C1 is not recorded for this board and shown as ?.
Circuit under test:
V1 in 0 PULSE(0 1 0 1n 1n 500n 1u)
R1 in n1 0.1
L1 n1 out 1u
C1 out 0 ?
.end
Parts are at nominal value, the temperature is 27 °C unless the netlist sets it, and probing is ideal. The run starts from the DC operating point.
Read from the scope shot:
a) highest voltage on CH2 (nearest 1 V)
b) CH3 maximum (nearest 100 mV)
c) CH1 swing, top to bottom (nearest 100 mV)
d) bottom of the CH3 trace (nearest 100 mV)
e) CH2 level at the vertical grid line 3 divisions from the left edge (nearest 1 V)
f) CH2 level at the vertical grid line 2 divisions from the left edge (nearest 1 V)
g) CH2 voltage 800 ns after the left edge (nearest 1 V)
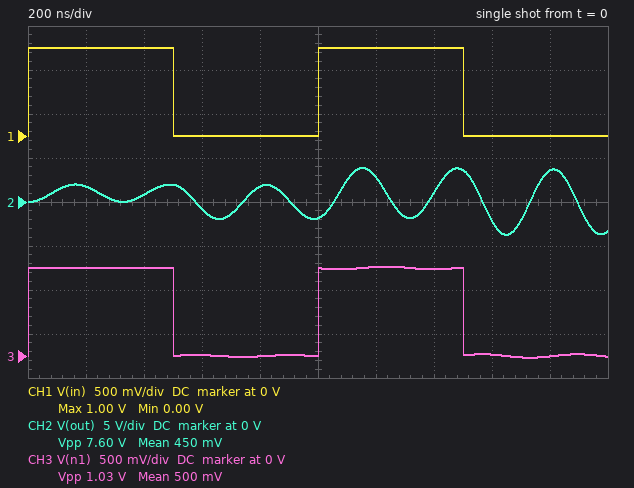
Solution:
4 V
1.0 V
1.0 V
0 V
-1 V
1 V
2 V
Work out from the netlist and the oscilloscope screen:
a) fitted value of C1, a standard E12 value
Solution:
2.7 nF
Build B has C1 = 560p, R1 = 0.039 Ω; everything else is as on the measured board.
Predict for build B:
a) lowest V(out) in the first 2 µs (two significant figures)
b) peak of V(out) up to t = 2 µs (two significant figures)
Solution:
-2.3 V
3.3 V
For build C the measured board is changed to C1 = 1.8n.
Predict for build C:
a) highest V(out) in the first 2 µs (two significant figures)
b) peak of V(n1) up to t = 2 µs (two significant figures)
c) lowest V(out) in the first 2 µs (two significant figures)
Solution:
2.0 V
1.0 V
-1.0 V
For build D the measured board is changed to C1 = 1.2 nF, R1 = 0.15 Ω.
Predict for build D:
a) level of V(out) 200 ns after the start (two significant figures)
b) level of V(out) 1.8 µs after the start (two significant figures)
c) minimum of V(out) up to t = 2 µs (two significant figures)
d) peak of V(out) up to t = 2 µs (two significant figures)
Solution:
150 mV
740 mV
-1.6 V
2.5 V
